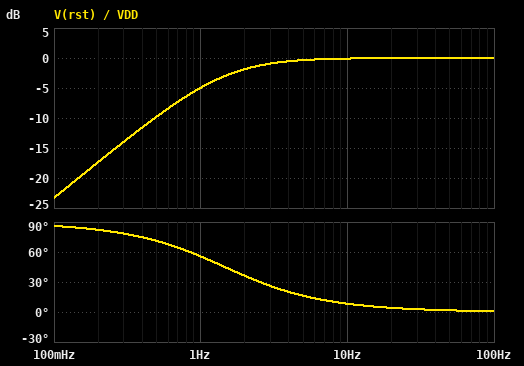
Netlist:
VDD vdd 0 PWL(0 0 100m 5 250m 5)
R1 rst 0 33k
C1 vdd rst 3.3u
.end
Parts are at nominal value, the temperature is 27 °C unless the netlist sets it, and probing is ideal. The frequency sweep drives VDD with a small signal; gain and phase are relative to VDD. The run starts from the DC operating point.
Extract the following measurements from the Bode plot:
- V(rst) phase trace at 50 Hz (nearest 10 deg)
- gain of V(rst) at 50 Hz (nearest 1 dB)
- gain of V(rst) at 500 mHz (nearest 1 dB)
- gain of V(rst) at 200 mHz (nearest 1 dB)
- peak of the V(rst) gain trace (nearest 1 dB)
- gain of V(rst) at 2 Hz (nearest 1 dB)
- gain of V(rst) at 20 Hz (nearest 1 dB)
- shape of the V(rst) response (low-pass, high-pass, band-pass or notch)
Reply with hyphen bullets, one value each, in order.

- 0 deg
- 0 dB
- -10 dB
- -17 dB
- 0 dB
- -2 dB
- 0 dB
- high-pass
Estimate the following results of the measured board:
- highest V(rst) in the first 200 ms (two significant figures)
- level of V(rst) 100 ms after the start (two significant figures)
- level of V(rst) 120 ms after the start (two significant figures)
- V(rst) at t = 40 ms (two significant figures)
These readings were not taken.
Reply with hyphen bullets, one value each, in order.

- 3.3 V
- 3.3 V
- 2.7 V
- 1.7 V
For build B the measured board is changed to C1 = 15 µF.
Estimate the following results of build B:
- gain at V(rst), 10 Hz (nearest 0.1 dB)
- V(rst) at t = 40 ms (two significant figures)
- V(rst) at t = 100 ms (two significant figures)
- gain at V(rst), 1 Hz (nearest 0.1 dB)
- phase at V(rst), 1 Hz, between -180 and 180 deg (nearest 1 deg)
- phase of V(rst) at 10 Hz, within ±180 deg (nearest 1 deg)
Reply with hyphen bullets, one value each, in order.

- 0 dB
- 1.9 V
- 4.5 V
- -0.4 dB
- 18 deg
- 2 deg
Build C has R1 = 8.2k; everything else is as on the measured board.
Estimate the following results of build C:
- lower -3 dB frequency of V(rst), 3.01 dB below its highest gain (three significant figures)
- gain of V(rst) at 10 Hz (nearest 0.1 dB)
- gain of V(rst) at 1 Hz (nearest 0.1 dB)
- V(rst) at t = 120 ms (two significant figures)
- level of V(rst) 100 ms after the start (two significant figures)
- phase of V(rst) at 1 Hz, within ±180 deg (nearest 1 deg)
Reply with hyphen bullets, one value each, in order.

- 5.88 Hz
- -1.3 dB
- -15.5 dB
- 630 mV
- 1.3 V
- 80 deg
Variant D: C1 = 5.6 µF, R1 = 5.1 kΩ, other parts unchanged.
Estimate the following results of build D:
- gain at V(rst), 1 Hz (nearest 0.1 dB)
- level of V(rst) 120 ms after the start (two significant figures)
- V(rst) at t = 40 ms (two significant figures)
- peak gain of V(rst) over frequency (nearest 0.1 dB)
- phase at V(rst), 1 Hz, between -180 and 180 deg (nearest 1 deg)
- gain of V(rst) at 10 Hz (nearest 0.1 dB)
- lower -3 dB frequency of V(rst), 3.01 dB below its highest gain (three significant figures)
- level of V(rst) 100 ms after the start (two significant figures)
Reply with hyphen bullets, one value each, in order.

- -15.1 dB
- 690 mV
- 1.1 V
- 0 dB
- 80 deg
- -1.2 dB
- 5.57 Hz
- 1.4 V
